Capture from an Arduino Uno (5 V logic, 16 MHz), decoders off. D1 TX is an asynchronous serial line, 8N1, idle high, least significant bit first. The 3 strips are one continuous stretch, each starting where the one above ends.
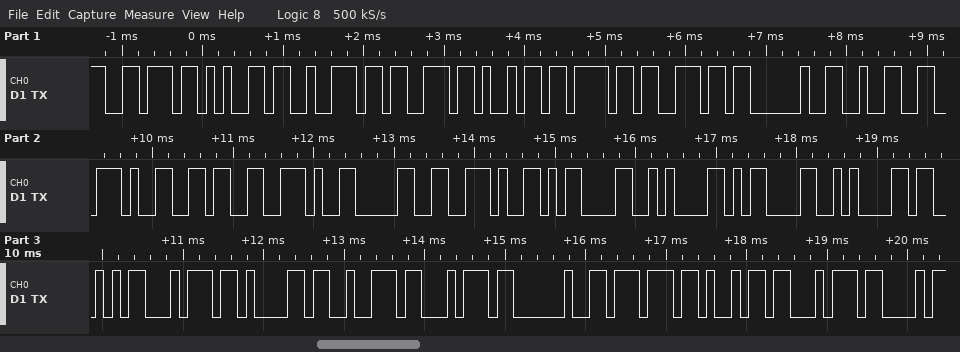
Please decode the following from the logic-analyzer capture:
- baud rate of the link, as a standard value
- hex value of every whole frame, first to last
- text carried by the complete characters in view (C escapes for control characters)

9600 baud
76 65 72 73 69 6F 6E 20 32 2E 36 2E 30 2E 0D 0A 0D 0A 53 74 61 72 74 20 77 69 74
"version 2.6.0.\r\n\r\nStart wit"
